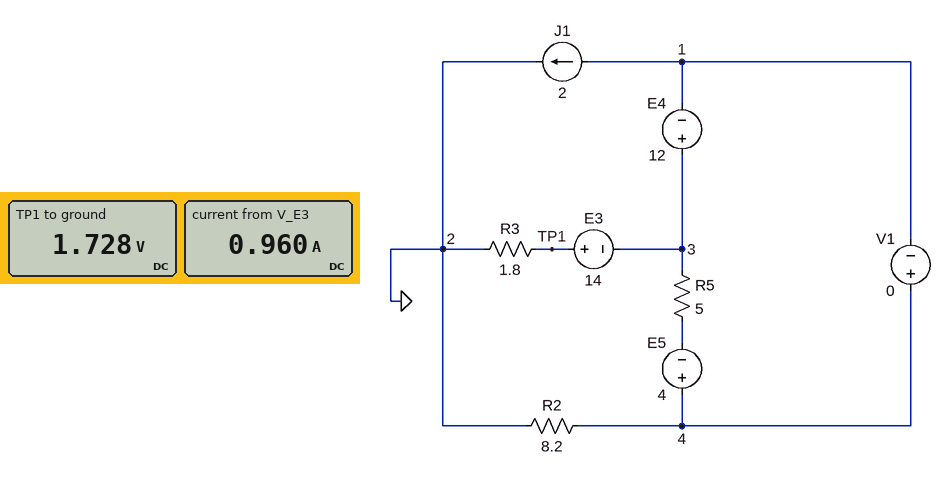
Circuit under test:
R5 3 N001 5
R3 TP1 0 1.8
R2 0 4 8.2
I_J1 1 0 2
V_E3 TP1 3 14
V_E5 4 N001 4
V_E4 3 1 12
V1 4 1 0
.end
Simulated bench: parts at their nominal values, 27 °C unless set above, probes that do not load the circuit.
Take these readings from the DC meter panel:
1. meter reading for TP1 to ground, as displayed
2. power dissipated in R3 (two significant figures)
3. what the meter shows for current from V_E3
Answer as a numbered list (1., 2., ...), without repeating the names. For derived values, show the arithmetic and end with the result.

1. 1.728 V
2. (1.728 V)^2 / 1.8 Ω = 1.7 W
3. 0.960 A
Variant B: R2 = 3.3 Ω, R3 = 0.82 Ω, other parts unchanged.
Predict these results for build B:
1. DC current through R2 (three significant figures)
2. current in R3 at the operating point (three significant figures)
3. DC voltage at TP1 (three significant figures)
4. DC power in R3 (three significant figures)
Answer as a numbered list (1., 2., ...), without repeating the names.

1. 6.71 A
2. 4.71 A
3. 3.86 V
4. 18.2 W
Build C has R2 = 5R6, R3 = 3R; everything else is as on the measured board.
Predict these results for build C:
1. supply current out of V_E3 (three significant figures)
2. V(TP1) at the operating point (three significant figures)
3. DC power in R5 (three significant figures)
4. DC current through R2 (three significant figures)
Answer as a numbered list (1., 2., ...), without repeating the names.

1. 1.72 A
2. 5.16 V
3. 51.2 W
4. 3.72 A
